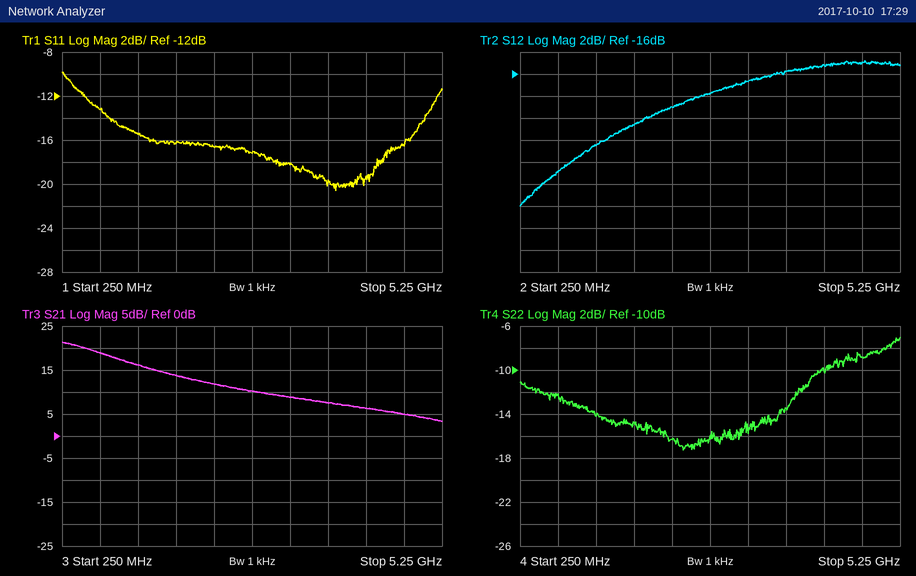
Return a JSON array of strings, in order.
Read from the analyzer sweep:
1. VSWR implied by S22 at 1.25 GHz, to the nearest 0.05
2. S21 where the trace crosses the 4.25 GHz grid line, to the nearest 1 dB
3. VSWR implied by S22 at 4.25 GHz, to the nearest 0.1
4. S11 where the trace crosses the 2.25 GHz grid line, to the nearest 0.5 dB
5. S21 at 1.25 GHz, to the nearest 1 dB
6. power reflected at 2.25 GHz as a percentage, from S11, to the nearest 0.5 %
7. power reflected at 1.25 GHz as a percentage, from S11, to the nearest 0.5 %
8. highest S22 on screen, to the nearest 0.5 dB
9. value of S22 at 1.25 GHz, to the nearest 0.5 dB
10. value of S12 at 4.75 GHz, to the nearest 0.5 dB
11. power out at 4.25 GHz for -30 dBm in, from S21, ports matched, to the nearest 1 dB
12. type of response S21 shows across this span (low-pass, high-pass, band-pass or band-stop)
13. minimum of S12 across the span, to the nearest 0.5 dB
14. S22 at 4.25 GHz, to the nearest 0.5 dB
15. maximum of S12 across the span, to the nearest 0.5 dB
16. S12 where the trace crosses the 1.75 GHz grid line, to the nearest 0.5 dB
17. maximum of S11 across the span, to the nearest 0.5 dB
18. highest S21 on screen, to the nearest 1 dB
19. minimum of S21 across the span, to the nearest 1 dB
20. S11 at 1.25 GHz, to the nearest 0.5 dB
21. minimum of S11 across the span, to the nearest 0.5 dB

["1.50", "6 dB", "1.9", "-16.5 dB", "16 dB", "2.0 %", "3.0 %", "-7.0 dB", "-14.0 dB", "-15.0 dB", "-24 dBm", "low-pass", "-28.0 dB", "-10.0 dB", "-15.0 dB", "-20.5 dB", "-10.0 dB", "21 dB", "3 dB", "-15.5 dB", "-20.5 dB"]
